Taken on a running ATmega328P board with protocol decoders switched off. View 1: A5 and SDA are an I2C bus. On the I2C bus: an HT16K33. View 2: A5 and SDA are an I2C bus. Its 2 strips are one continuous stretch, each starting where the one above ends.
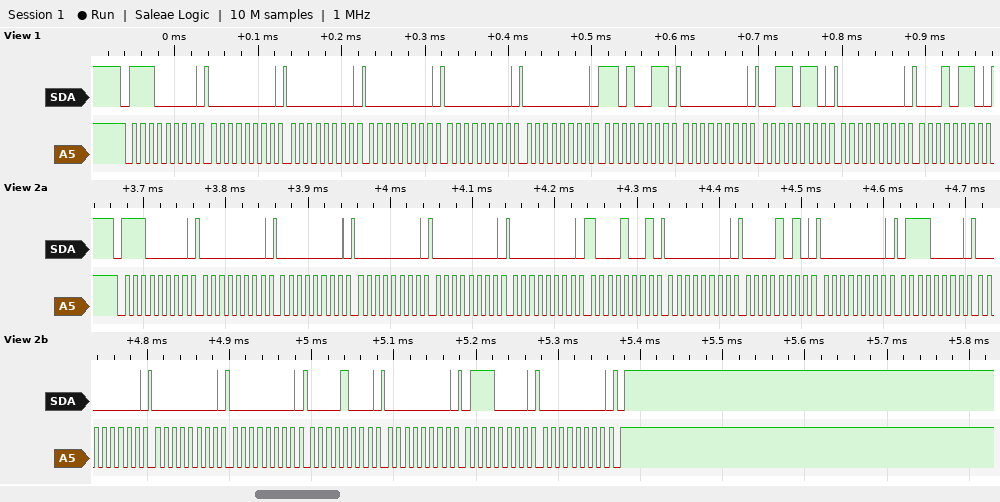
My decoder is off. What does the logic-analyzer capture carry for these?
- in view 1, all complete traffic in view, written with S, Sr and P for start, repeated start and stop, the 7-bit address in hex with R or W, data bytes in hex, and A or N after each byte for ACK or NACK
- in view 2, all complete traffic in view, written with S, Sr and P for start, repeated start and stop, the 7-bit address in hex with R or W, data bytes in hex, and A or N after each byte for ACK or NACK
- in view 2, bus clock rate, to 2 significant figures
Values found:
S 70W A 00 A 00 A 00 A 00 A 00 A D3 A 00 A 36 A 00 A 16 A
S 70W A 00 A 00 A 00 A 00 A 00 A 89 A 00 A 0A A 00 A 70 A 00 A 00 A 00 A 08 A 00 A 70 A 00 A P
100 kHz
